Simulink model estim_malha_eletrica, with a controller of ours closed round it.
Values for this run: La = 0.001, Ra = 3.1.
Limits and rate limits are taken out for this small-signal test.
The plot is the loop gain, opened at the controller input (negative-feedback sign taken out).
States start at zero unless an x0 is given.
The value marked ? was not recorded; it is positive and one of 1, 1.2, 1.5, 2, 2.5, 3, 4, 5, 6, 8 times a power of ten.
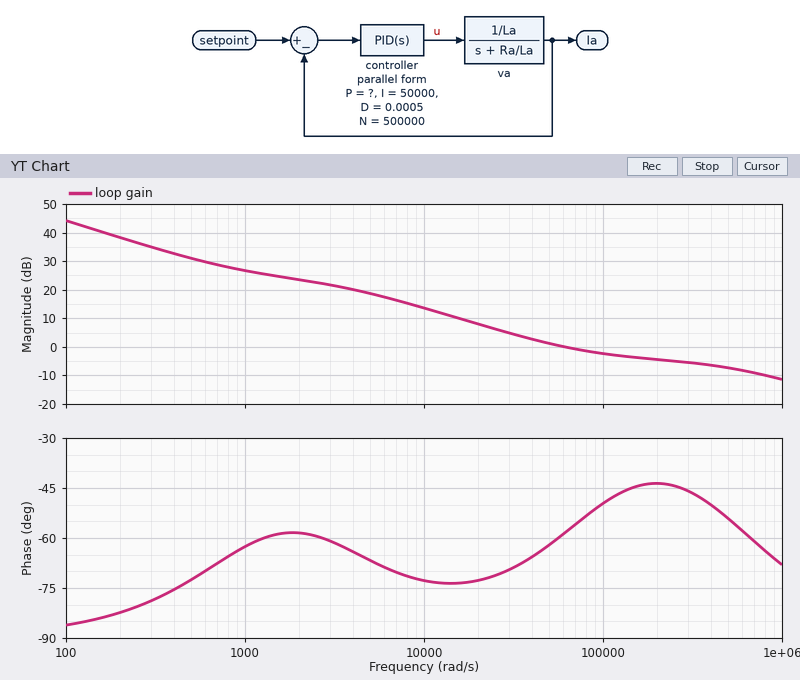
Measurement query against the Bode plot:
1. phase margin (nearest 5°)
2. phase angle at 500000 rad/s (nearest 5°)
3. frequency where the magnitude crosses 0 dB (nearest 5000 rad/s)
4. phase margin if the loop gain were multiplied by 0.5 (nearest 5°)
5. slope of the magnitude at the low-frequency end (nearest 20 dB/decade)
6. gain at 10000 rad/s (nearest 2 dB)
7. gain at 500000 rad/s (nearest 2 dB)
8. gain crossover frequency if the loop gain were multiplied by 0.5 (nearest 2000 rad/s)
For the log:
120°
-55°
60000 rad/s
110°
-20 dB/decade
14 dB
-8 dB
26000 rad/s
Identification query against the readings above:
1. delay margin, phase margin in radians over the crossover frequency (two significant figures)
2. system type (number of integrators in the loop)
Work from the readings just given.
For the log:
0.000035 s
1
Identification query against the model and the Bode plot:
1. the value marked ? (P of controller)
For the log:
50
